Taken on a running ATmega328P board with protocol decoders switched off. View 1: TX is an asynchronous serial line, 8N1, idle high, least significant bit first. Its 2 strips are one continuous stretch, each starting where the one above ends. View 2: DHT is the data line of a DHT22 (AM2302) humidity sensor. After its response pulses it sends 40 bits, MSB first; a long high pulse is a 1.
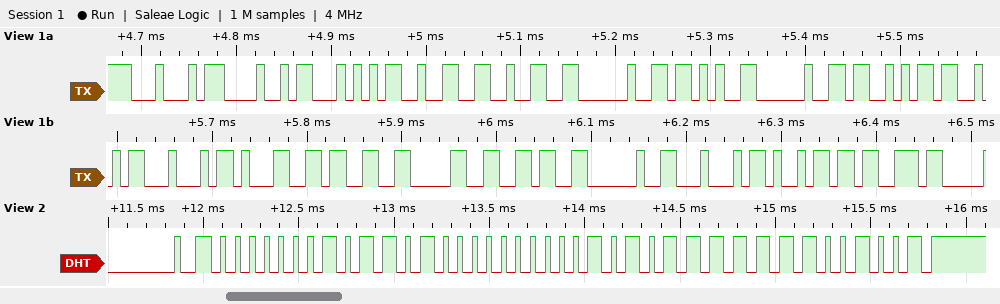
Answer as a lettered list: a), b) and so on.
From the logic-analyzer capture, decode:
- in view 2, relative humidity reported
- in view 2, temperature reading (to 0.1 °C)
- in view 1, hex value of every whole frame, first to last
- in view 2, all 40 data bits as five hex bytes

a) 36.0 %
b) 35.1 °C
c) 44 48 54 32 32 20 2B 20 53 53 44 31 33 30 36 20 44 69 73
d) 01 68 01 5F C9
